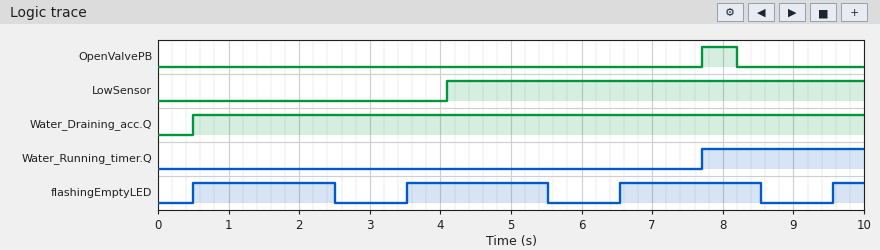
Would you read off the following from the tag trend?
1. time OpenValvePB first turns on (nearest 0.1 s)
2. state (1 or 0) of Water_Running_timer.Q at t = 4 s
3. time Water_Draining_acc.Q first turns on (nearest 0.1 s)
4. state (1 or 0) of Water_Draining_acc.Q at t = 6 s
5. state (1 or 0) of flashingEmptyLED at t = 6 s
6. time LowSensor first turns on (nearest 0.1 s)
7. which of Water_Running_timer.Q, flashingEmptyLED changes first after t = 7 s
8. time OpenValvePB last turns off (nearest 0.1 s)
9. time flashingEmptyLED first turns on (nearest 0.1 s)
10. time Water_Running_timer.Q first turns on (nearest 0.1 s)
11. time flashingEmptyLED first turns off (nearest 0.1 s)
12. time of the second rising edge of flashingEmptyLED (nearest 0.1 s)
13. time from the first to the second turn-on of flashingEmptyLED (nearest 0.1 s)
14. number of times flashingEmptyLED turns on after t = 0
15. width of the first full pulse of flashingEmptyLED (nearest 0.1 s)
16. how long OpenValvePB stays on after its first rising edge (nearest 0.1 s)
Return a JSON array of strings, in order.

["7.7 s", "0", "0.5 s", "1", "0", "4.1 s", "Water_Running_timer.Q", "8.2 s", "0.5 s", "7.7 s", "2.5 s", "3.5 s", "3.0 s", "4", "2.0 s", "0.5 s"]
